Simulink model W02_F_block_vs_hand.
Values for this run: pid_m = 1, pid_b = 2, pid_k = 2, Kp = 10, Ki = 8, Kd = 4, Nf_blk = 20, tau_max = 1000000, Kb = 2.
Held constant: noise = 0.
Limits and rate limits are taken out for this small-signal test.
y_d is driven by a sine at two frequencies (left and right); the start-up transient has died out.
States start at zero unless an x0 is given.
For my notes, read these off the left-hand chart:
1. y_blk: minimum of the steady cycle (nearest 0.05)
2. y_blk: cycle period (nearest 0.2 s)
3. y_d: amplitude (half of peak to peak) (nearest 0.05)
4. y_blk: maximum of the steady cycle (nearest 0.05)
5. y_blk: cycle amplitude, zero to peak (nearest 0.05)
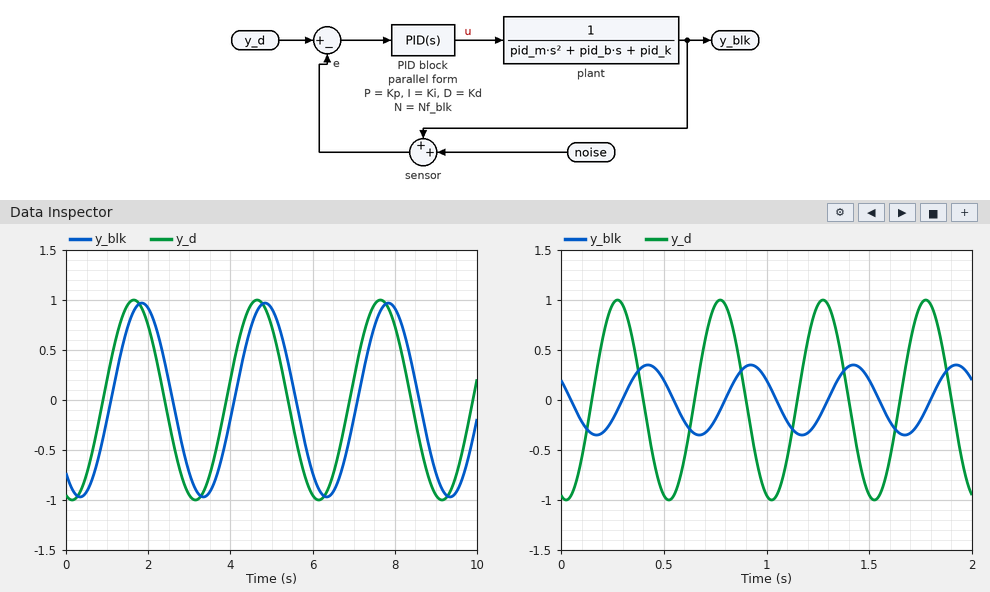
-0.95
3.0 s
1.00
0.95
0.95
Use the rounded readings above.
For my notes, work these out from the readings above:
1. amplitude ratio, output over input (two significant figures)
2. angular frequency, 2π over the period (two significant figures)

0.95
2.1 rad/s
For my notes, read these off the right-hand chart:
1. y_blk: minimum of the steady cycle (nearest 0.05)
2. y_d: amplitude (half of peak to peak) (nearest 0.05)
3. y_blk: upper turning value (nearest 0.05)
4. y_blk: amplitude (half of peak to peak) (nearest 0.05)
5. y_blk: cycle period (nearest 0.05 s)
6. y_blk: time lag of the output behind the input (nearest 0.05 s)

-0.35
1.00
0.35
0.35
0.50 s
0.15 s
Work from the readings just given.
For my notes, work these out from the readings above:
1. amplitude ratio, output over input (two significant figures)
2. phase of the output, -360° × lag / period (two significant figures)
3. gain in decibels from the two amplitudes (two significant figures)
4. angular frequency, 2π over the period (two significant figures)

0.35
-110°
-9.1 dB
13 rad/s
